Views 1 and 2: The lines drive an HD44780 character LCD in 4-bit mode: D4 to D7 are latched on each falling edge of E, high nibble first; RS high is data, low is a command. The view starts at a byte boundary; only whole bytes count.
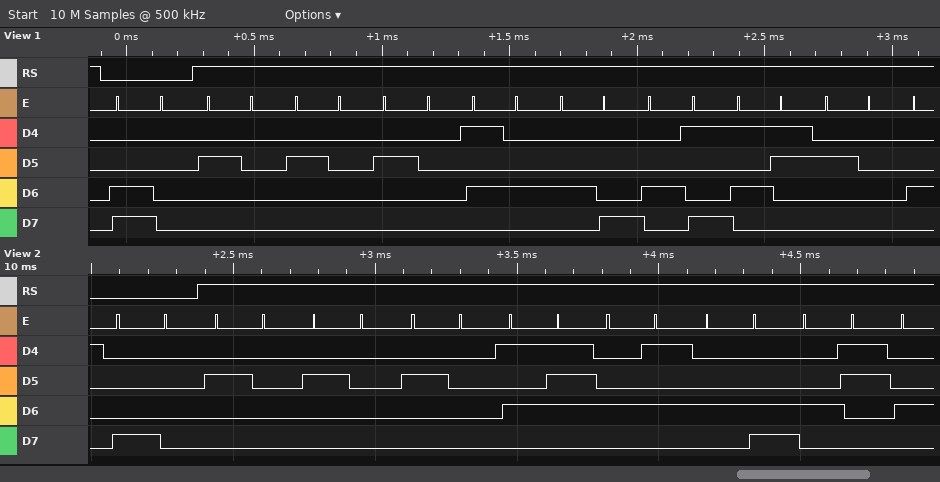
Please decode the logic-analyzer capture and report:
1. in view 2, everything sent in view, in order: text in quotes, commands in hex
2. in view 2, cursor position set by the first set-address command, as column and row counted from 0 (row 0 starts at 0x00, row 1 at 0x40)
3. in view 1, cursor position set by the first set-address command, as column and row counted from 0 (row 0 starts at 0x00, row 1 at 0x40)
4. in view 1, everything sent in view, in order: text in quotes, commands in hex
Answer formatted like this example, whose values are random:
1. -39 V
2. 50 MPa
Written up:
1. 0x80 "   WELC"
2. column 0, row 0
3. column 0, row 1
4. 0xC0 "   THIS "
